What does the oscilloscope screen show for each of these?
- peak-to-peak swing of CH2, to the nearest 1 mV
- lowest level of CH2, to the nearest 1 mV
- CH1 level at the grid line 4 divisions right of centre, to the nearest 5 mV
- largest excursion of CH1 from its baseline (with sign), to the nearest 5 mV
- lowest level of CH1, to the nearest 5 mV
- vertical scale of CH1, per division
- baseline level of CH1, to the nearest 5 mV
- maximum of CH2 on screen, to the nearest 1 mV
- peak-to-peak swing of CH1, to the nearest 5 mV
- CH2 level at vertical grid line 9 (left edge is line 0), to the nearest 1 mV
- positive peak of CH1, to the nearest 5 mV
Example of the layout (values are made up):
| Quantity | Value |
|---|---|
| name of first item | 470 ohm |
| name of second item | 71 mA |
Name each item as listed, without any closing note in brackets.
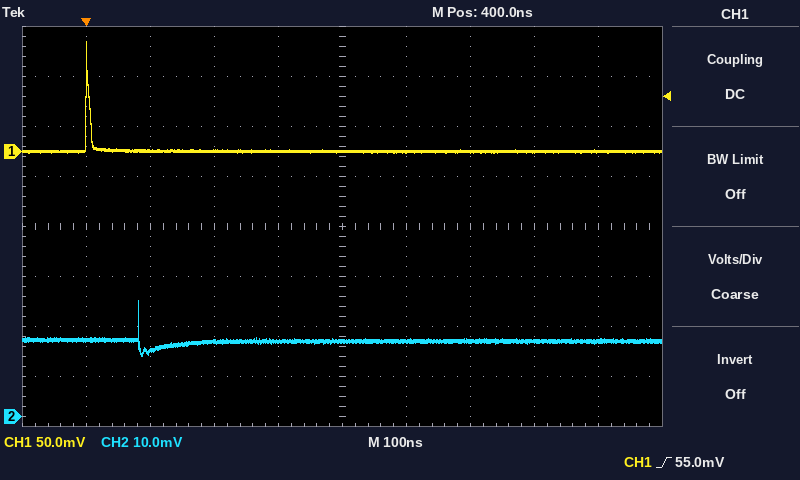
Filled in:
| Quantity | Value |
|---|---|
| peak-to-peak swing of CH2, to the nearest 1 mV | 11 mV |
| lowest level of CH2, to the nearest 1 mV | 12 mV |
| CH1 level at the grid line 4 divisions right of centre, to the nearest 5 mV | 0 mV |
| largest excursion of CH1 from its baseline (with sign), to the nearest 5 mV | +110 mV |
| lowest level of CH1, to the nearest 5 mV | 0 mV |
| vertical scale of CH1, per division | 50 mV |
| baseline level of CH1, to the nearest 5 mV | 0 mV |
| maximum of CH2 on screen, to the nearest 1 mV | 23 mV |
| peak-to-peak swing of CH1, to the nearest 5 mV | 110 mV |
| CH2 level at vertical grid line 9 (left edge is line 0), to the nearest 1 mV | 15 mV |
| positive peak of CH1, to the nearest 5 mV | 110 mV |
